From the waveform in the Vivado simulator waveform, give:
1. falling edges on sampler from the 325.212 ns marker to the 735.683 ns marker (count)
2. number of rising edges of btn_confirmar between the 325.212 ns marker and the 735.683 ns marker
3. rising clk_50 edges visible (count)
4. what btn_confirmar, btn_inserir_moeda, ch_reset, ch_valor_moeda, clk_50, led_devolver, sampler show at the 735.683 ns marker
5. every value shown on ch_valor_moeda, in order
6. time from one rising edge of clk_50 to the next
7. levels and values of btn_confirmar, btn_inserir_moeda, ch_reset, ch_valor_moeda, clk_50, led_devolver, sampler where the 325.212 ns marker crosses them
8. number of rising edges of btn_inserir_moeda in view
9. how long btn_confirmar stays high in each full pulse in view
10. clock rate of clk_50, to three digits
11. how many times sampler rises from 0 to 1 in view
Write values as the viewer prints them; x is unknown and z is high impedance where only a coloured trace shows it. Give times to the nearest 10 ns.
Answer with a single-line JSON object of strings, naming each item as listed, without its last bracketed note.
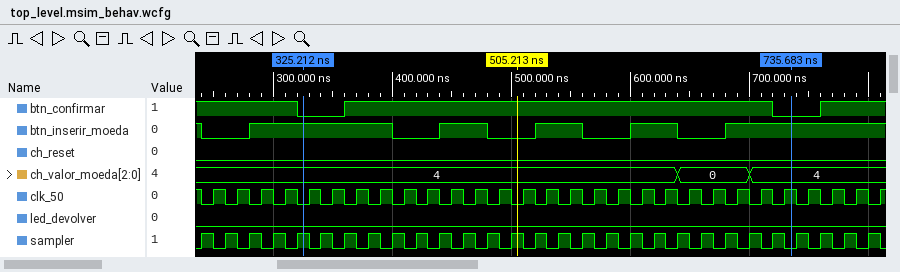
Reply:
{"falling edges on sampler from the 325.212 ns marker to the 735.683 ns marker": "21", "number of rising edges of btn_confirmar between the 325.212 ns marker and the 735.683 ns marker": "1", "rising clk_50 edges visible": "29", "what btn_confirmar, btn_inserir_moeda, ch_reset, ch_valor_moeda, clk_50, led_devolver, sampler show at the 735.683 ns marker": "btn_confirmar=0, btn_inserir_moeda=1, ch_reset=0, ch_valor_moeda=4, clk_50=1, led_devolver=0, sampler=0", "every value shown on ch_valor_moeda, in order": "4, 0, 4", "time from one rising edge of clk_50 to the next": "20 ns", "levels and values of btn_confirmar, btn_inserir_moeda, ch_reset, ch_valor_moeda, clk_50, led_devolver, sampler where the 325.212 ns marker crosses them": "btn_confirmar=0, btn_inserir_moeda=1, ch_reset=0, ch_valor_moeda=4, clk_50=0, led_devolver=0, sampler=1", "number of rising edges of btn_inserir_moeda in view": "5", "how long btn_confirmar stays high in each full pulse in view": "360 ns", "clock rate of clk_50, to three digits": "50.0 MHz", "how many times sampler rises from 0 to 1 in view": "29"}
